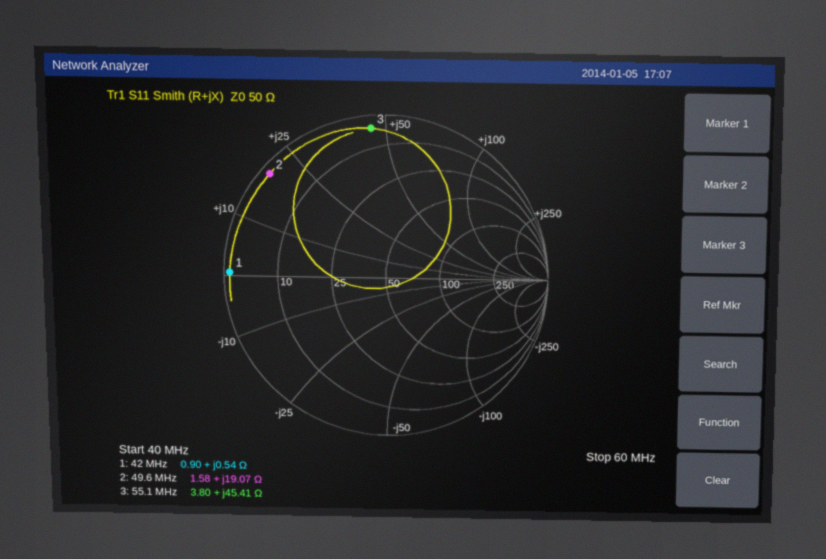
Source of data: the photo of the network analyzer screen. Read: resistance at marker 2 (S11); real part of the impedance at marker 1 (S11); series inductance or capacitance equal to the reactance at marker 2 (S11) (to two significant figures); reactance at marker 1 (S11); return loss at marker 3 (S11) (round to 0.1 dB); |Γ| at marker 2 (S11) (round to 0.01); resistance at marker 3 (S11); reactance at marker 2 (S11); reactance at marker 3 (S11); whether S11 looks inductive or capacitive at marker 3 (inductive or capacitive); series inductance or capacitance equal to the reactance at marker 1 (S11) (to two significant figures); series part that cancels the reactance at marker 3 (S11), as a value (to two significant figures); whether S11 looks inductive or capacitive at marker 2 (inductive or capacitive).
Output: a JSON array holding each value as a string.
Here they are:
["1.58 Ω", "0.90 Ω", "61 nH", "+0.54 Ω", "0.7 dB", "0.95", "3.80 Ω", "+19.07 Ω", "+45.41 Ω", "inductive", "2.0 nH", "64 pF", "inductive"]
